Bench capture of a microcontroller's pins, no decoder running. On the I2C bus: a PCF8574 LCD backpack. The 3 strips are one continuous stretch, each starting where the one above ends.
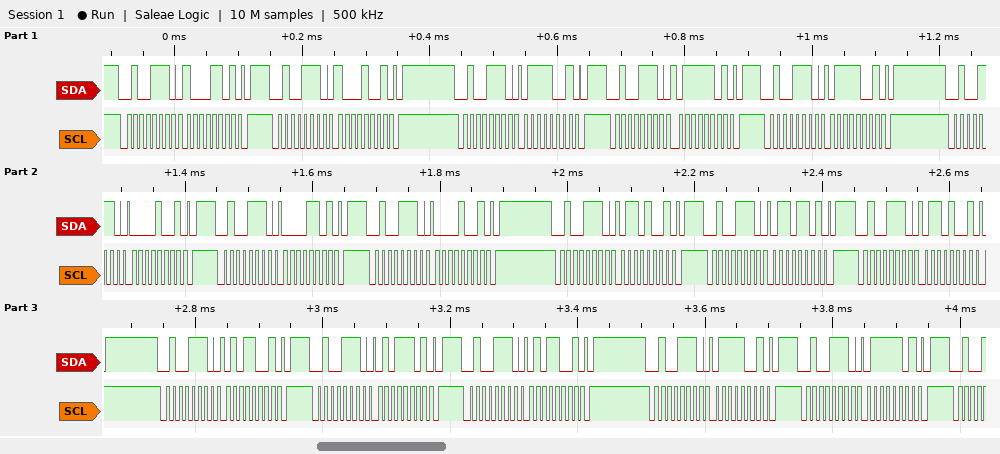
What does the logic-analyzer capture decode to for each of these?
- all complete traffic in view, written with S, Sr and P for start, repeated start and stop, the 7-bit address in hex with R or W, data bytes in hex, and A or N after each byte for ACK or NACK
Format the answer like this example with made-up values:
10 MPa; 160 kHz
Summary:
S 27W A 8D A P S 27W A 89 A P S 27W A 79 A P S 27W A 7D A P S 27W A 79 A P S 27W A 09 A P S 27W A 0D A P S 27W A 09 A P S 27W A 69 A P S 27W A 6D A P S 27W A 69 A P S 27W A 59 A P S 27W A 5D A P S 27W A 59 A P S 27W A 79 A P S 27W A 7D A P
